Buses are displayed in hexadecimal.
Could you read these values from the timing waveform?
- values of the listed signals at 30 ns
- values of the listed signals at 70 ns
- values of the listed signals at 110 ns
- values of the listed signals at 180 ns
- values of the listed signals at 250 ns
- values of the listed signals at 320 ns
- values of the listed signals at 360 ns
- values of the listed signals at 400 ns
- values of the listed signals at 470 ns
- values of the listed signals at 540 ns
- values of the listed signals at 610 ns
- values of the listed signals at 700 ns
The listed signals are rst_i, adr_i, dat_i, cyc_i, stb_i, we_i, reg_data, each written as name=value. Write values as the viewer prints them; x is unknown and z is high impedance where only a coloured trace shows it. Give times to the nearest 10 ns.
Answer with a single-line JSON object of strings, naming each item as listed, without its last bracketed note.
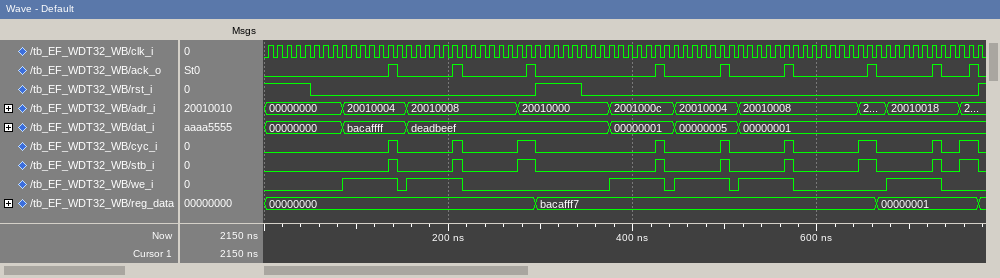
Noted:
{"values of the listed signals at 30 ns": "rst_i=1, adr_i=00000000, dat_i=00000000, cyc_i=0, stb_i=0, we_i=0, reg_data=00000000", "values of the listed signals at 70 ns": "rst_i=0, adr_i=00000000, dat_i=00000000, cyc_i=0, stb_i=0, we_i=0, reg_data=00000000", "values of the listed signals at 110 ns": "rst_i=0, adr_i=20010004, dat_i=bacaffff, cyc_i=0, stb_i=0, we_i=1, reg_data=00000000", "values of the listed signals at 180 ns": "rst_i=0, adr_i=20010008, dat_i=deadbeef, cyc_i=0, stb_i=0, we_i=1, reg_data=00000000", "values of the listed signals at 250 ns": "rst_i=0, adr_i=20010008, dat_i=deadbeef, cyc_i=0, stb_i=0, we_i=0, reg_data=00000000", "values of the listed signals at 320 ns": "rst_i=1, adr_i=20010000, dat_i=deadbeef, cyc_i=0, stb_i=0, we_i=0, reg_data=bacafff7", "values of the listed signals at 360 ns": "rst_i=0, adr_i=20010000, dat_i=deadbeef, cyc_i=0, stb_i=0, we_i=0, reg_data=bacafff7", "values of the listed signals at 400 ns": "rst_i=0, adr_i=2001000c, dat_i=00000001, cyc_i=0, stb_i=0, we_i=1, reg_data=bacafff7", "values of the listed signals at 470 ns": "rst_i=0, adr_i=20010004, dat_i=00000005, cyc_i=0, stb_i=0, we_i=1, reg_data=bacafff7", "values of the listed signals at 540 ns": "rst_i=0, adr_i=20010008, dat_i=00000001, cyc_i=0, stb_i=0, we_i=1, reg_data=bacafff7", "values of the listed signals at 610 ns": "rst_i=0, adr_i=20010008, dat_i=00000001, cyc_i=0, stb_i=0, we_i=0, reg_data=bacafff7", "values of the listed signals at 700 ns": "rst_i=0, adr_i=20010018, dat_i=00000001, cyc_i=0, stb_i=0, we_i=1, reg_data=00000001"}
